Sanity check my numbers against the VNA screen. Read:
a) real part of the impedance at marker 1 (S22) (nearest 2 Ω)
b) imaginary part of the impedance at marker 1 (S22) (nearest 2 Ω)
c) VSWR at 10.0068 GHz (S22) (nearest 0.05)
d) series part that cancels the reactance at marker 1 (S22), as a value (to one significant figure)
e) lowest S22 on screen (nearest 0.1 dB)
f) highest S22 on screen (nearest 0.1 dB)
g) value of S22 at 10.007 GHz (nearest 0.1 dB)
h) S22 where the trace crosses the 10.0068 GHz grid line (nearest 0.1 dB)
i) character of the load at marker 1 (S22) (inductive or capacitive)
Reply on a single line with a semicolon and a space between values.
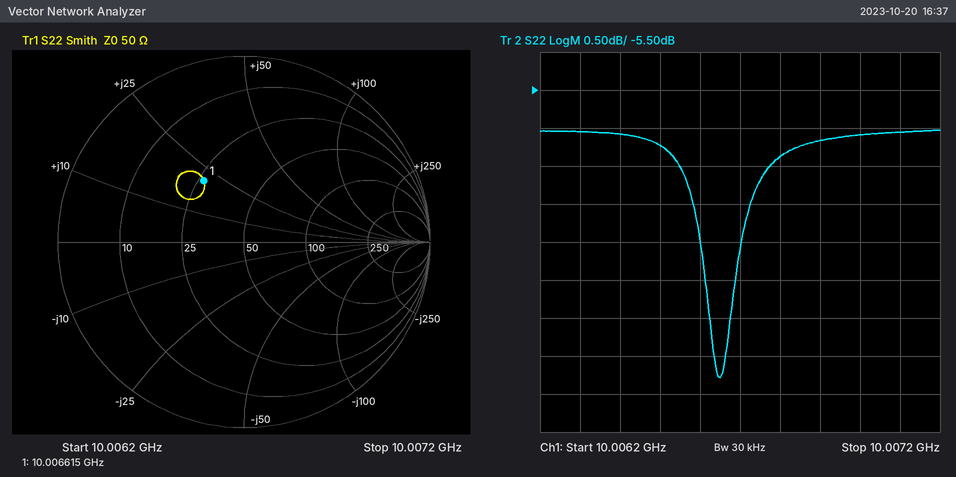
26 Ω; +20 Ω; 2.85; 800 fF; -9.3 dB; -6.0 dB; -6.1 dB; -6.4 dB; inductive
